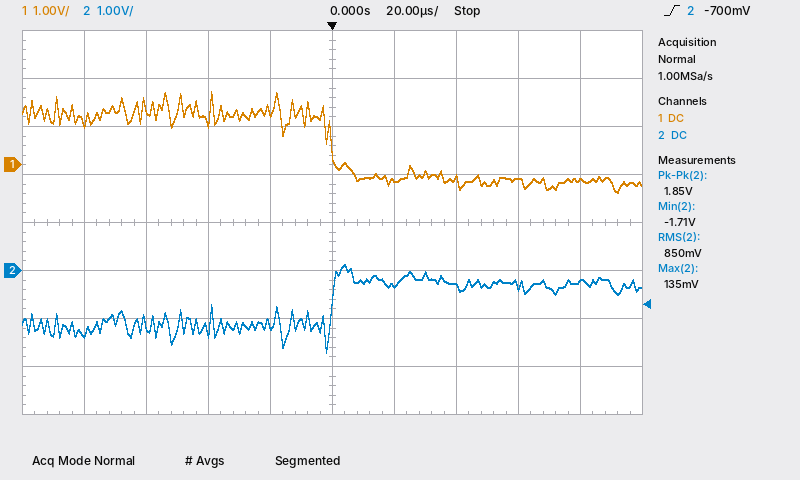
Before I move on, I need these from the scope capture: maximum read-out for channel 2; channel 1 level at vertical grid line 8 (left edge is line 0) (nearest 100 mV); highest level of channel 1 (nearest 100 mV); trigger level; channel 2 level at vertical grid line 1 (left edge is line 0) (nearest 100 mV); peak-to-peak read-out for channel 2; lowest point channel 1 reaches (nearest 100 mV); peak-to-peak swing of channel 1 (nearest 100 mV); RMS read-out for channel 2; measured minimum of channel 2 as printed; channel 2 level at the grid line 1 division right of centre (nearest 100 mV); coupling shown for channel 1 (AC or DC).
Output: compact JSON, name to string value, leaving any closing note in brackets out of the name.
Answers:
{"maximum read-out for channel 2": "135 mV", "channel 1 level at vertical grid line 8 (left edge is line 0)": "-300 mV", "highest level of channel 1": "1.5 V", "trigger level": "-700 mV", "channel 2 level at vertical grid line 1 (left edge is line 0)": "-1.3 V", "peak-to-peak read-out for channel 2": "1.85 V", "lowest point channel 1 reaches": "-600 mV", "peak-to-peak swing of channel 1": "2.1 V", "RMS read-out for channel 2": "850 mV", "measured minimum of channel 2 as printed": "-1.71 V", "channel 2 level at the grid line 1 division right of centre": "-300 mV", "coupling shown for channel 1": "DC"}
